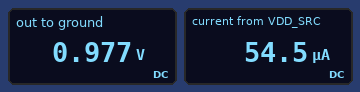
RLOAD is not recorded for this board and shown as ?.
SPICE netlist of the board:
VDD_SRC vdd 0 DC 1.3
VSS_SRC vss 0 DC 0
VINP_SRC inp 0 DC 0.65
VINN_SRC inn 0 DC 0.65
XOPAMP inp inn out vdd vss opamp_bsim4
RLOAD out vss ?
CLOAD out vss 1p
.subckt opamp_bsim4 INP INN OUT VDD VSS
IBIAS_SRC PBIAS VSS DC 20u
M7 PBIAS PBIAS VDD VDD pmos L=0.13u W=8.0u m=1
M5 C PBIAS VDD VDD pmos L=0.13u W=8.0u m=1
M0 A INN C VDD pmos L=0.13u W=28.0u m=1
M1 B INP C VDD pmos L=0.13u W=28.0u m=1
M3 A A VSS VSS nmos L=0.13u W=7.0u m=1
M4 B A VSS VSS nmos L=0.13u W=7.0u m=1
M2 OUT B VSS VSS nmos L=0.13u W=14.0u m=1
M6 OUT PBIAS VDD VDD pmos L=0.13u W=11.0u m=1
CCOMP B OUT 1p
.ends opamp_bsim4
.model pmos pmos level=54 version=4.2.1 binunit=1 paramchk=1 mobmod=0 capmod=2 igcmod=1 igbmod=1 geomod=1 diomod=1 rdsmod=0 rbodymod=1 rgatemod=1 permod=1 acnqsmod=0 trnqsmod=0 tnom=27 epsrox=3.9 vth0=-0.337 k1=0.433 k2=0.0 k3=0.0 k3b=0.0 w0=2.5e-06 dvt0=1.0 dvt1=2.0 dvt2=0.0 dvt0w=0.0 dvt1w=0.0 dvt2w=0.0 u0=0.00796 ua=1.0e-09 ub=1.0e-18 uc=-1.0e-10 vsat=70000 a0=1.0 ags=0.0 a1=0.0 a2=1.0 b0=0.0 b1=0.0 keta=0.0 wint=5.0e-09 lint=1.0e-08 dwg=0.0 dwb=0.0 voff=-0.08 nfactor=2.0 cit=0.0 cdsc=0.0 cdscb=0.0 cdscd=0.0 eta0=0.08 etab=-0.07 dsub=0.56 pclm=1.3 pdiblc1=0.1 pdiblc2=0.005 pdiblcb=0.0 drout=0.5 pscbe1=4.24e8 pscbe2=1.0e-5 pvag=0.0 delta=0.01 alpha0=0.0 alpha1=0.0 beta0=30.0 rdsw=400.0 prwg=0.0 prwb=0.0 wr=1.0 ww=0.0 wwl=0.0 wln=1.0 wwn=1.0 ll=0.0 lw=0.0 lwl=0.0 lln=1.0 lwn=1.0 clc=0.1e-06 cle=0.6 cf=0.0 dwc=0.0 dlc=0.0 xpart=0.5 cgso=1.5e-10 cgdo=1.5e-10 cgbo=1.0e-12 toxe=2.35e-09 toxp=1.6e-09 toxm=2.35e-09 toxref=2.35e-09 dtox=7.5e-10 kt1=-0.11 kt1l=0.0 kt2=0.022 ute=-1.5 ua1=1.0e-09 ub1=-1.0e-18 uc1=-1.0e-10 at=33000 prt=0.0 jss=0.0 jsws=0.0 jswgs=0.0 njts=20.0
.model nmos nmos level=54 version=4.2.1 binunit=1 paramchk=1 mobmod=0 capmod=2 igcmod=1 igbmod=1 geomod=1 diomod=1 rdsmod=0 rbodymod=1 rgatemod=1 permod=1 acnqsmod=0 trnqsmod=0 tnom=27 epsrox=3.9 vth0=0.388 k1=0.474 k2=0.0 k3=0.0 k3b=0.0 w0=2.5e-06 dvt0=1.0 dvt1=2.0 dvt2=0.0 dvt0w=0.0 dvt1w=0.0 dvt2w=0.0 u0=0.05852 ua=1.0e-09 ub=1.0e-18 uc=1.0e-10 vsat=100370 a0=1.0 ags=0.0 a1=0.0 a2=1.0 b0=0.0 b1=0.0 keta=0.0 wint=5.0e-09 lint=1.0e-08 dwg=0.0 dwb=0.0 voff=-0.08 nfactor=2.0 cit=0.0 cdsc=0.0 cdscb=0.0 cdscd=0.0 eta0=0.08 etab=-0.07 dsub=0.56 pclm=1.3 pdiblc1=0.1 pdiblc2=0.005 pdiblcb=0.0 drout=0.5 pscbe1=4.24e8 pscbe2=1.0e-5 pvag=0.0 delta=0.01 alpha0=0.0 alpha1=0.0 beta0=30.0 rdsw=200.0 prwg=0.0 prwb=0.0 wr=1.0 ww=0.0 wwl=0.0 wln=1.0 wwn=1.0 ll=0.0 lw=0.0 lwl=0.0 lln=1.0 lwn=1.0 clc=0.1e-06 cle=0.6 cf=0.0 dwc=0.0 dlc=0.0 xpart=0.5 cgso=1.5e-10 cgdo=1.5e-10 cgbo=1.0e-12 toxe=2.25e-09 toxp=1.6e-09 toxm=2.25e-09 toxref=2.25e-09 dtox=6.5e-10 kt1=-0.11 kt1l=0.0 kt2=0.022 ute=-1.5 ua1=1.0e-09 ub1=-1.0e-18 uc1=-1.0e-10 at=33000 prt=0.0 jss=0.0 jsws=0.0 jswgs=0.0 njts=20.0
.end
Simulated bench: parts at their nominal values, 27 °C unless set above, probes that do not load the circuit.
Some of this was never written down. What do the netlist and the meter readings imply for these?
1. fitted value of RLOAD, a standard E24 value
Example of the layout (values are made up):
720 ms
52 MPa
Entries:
200 kΩ
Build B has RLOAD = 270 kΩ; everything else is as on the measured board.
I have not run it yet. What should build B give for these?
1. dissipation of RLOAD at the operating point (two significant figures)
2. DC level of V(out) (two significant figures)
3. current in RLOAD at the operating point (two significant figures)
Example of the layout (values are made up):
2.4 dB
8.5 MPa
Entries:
3.8 µW
1.0 V
3.8 µA
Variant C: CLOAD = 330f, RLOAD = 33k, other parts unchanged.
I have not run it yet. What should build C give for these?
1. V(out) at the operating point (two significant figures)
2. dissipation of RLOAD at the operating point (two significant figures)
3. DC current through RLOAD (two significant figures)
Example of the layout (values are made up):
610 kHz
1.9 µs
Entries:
570 mV
9.7 µW
17 µA
